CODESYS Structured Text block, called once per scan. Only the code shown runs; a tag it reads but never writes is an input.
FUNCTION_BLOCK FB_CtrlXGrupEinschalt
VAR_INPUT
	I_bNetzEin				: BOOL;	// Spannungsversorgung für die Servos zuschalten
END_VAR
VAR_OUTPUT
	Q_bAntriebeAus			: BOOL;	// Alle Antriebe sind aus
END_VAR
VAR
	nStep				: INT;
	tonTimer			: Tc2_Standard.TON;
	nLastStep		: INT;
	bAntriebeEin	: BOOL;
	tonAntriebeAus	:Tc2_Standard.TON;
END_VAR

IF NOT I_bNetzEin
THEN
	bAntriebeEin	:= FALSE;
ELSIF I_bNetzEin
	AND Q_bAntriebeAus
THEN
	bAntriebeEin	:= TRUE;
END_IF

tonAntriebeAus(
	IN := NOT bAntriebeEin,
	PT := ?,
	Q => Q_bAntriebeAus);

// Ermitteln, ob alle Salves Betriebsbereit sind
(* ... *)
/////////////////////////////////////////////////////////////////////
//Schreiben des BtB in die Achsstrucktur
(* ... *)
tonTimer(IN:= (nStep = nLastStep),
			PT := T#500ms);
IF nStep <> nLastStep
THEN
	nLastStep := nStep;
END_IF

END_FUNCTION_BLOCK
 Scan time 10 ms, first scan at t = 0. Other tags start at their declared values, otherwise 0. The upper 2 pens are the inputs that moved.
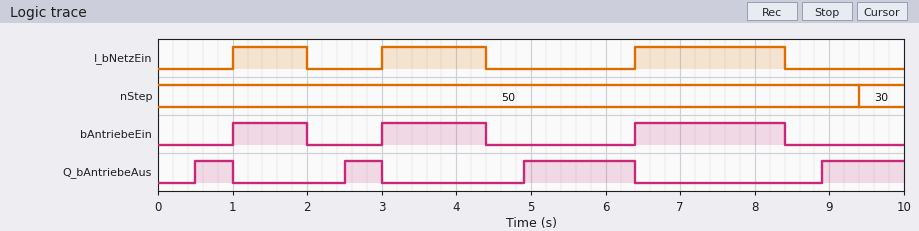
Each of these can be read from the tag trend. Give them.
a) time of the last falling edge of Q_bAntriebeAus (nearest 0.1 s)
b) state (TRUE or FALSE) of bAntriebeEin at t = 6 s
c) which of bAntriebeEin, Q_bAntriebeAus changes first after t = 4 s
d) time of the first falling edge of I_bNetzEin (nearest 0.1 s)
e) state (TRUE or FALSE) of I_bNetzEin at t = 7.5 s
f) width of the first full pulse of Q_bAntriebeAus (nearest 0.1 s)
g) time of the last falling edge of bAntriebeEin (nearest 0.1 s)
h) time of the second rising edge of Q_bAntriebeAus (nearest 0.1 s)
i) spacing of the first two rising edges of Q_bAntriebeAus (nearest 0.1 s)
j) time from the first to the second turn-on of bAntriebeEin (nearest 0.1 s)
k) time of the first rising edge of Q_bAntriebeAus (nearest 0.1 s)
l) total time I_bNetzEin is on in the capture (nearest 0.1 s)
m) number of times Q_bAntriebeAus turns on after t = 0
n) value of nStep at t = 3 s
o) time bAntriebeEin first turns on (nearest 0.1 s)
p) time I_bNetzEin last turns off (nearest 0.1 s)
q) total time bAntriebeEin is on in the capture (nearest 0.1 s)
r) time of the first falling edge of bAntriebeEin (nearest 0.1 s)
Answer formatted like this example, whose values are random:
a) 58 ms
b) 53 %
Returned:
a) 6.4 s
b) FALSE
c) bAntriebeEin
d) 2.0 s
e) TRUE
f) 0.5 s
g) 8.4 s
h) 2.5 s
i) 2.0 s
j) 2.0 s
k) 0.5 s
l) 4.4 s
m) 4
n) 50
o) 1.0 s
p) 8.4 s
q) 4.4 s
r) 2.0 s
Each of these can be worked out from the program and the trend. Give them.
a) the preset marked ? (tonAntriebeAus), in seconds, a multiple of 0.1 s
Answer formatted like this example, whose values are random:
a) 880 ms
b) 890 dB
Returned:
a) 0.5 s
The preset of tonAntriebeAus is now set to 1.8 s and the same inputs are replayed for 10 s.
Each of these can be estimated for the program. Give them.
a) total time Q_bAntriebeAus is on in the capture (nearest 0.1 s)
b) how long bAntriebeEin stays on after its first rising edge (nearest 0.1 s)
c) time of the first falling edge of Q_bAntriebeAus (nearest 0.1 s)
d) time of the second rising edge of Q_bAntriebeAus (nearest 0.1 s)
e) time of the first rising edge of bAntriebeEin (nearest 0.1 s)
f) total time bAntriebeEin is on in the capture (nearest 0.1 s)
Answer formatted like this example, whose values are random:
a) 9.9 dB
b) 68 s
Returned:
a) 0.2 s
b) 0.2 s
c) 1.8 s
d) 3.8 s
e) 1.8 s
f) 2.8 s
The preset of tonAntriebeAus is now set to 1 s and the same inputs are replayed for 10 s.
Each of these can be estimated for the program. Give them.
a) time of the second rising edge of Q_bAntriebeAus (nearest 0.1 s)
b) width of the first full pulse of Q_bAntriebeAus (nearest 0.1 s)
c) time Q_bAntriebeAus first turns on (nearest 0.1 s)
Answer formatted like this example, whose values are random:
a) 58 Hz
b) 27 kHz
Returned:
a) 3.0 s
b) 0.0 s
c) 1.0 s
